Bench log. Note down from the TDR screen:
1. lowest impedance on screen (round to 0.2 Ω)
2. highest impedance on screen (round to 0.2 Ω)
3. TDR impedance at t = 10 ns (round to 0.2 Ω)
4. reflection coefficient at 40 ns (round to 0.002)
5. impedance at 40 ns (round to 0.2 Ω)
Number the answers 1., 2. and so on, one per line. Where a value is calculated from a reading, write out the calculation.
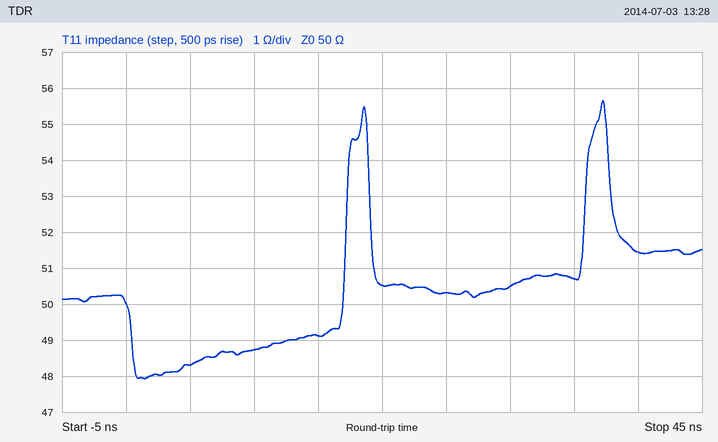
1. 48.0 Ω
2. 55.6 Ω
3. 48.8 Ω
4. (51.4 − 50)/(51.4 + 50) ≈ +0.014
5. 51.4 Ω
